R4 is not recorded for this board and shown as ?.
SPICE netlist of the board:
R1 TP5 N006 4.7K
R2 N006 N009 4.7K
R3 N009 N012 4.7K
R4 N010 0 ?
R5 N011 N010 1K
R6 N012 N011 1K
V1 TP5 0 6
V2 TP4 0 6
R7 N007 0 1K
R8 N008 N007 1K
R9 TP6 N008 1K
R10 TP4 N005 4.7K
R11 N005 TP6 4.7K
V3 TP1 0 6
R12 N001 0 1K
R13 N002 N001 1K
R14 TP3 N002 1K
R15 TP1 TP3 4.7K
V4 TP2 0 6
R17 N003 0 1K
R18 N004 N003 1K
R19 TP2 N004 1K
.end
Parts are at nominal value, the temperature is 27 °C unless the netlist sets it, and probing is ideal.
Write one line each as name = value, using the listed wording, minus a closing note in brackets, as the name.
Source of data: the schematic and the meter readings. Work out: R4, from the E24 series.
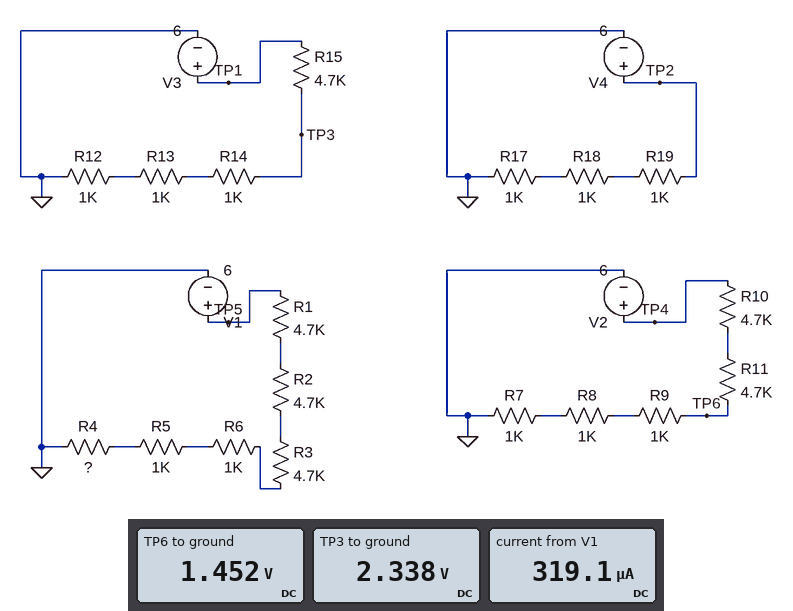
R4, from the E24 series = 2.7 kΩ
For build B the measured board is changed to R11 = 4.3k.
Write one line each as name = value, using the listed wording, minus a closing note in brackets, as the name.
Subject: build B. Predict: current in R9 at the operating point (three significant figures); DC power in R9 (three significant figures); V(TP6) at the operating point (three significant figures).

current in R9 at the operating point = 500 µA
DC power in R9 = 250 µW
V(TP6) at the operating point = 1.50 V
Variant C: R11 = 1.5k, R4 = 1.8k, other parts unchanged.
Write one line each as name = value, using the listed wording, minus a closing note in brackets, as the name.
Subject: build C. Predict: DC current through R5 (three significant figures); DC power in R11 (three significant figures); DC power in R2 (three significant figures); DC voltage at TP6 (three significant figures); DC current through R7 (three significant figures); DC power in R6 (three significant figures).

DC current through R5 = 335 µA
DC power in R11 = 638 µW
DC power in R2 = 528 µW
DC voltage at TP6 = 1.96 V
DC current through R7 = 652 µA
DC power in R6 = 112 µW
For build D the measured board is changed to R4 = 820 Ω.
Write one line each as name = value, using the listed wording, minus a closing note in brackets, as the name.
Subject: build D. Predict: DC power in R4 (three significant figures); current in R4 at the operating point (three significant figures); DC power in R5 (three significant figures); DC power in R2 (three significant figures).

DC power in R4 = 103 µW
current in R4 at the operating point = 355 µA
DC power in R5 = 126 µW
DC power in R2 = 591 µW
